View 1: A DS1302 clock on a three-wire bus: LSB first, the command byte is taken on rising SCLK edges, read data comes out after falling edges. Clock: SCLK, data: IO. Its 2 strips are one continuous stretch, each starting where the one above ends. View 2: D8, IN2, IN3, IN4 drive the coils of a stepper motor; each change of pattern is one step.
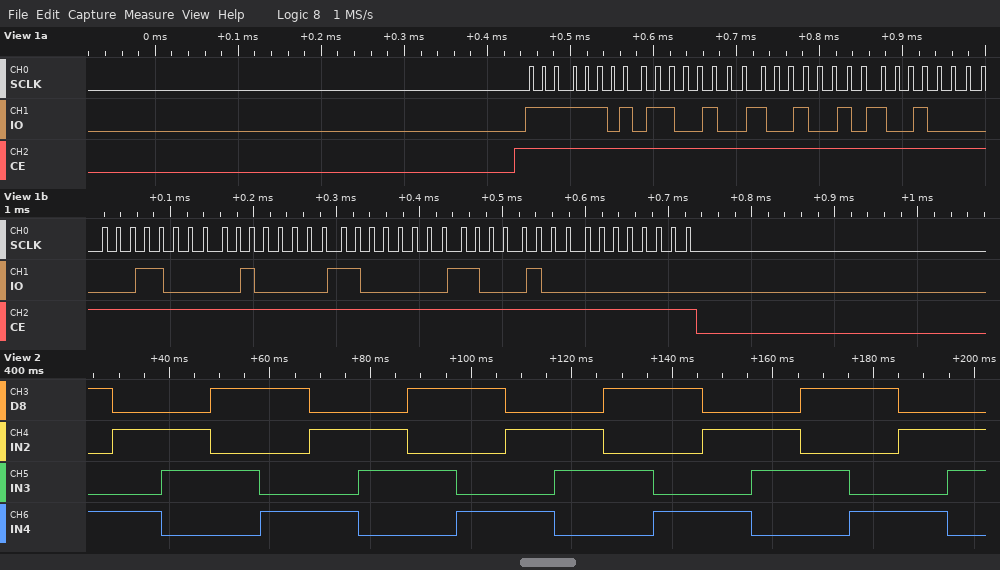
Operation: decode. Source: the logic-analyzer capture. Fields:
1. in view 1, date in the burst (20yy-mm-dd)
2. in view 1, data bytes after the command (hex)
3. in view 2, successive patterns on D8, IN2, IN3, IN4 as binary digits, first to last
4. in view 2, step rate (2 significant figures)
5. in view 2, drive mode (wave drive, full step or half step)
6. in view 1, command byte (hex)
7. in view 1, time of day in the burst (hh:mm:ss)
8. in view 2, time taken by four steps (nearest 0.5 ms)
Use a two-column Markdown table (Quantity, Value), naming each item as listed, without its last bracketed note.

| Quantity | Value |
|---|---|
| in view 1, date in the burst | 2023-04-18 |
| in view 1, data bytes after the command | 26 49 09 18 04 03 23 00 |
| in view 2, successive patterns on D8, IN2, IN3, IN4 as binary digits, first to last | 1001 0101 0110 1010 1001 0101 0110 1010 1001 0101 0110 1010 1001 0101 0110 1010 1001 0101 0110 |
| in view 2, step rate | 100 steps/s |
| in view 2, drive mode | full step |
| in view 1, command byte | 0xBF |
| in view 1, time of day in the burst | 09:49:26 |
| in view 2, time taken by four steps | 39.0 ms |
